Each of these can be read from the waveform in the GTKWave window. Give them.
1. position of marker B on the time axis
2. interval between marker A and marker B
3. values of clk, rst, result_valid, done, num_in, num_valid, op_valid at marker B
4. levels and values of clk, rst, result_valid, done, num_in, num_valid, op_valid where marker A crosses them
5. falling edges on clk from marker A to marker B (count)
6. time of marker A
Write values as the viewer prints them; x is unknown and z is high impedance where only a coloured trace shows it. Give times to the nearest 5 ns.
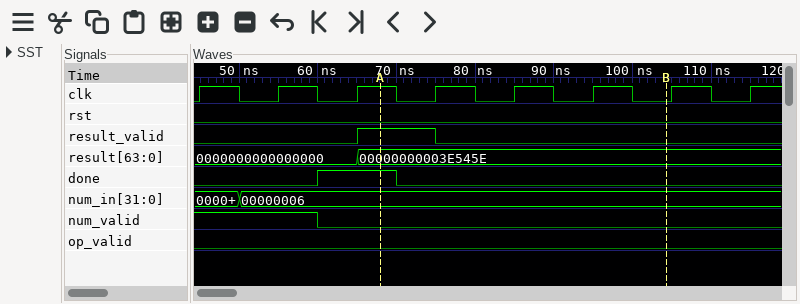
105 ns
35 ns
clk=0, rst=0, result_valid=0, done=0, num_in=00000006, num_valid=0, op_valid=0
clk=1, rst=0, result_valid=1, done=1, num_in=00000006, num_valid=0, op_valid=0
4
70 ns
